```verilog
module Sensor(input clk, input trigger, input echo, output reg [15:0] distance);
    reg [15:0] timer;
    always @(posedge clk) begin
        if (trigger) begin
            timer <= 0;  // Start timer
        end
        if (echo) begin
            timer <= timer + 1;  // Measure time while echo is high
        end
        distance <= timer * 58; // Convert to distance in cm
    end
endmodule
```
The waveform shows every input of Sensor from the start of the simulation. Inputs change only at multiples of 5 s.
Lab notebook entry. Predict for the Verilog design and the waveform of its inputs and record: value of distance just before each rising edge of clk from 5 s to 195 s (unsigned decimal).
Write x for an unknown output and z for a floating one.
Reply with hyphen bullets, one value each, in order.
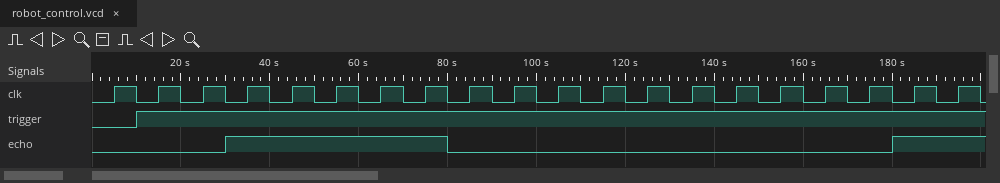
- x, x, x, 0, 0, 58, 116, 174, 232, 290, 0, 0, 0, 0, 0, 0, 0, 0, 0, 0
